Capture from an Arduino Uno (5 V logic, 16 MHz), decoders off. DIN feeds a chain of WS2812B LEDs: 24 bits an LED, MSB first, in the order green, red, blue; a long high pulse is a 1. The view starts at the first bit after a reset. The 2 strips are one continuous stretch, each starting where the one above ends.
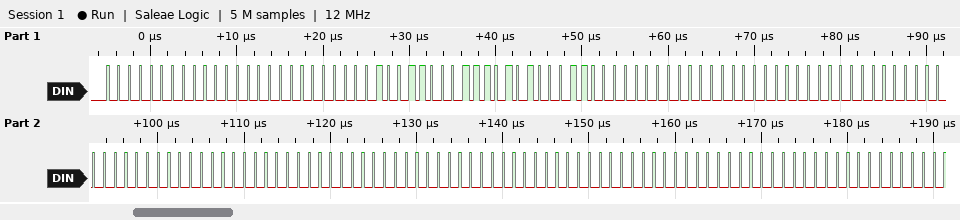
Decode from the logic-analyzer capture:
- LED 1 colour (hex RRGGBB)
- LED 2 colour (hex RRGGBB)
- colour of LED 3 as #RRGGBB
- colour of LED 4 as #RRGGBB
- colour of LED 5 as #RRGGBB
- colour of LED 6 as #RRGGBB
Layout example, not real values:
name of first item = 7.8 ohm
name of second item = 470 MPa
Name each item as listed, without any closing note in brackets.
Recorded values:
LED 1 colour = #000000
LED 2 colour = #754C18
colour of LED 3 as #RRGGBB = #000000
colour of LED 4 as #RRGGBB = #000000
colour of LED 5 as #RRGGBB = #000000
colour of LED 6 as #RRGGBB = #000000
